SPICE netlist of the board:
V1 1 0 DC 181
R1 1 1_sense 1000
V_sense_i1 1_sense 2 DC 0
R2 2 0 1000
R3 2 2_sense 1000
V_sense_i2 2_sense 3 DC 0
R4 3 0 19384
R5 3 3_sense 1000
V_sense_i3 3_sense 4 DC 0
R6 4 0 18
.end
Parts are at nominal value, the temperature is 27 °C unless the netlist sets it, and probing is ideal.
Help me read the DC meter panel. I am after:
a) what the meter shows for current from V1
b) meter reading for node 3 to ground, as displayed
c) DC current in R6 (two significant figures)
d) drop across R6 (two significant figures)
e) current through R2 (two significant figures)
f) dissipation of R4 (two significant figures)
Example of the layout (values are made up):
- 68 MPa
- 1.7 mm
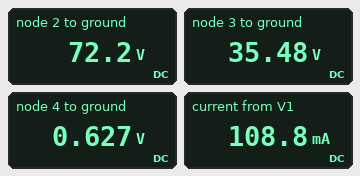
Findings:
- 108.8 mA
- 35.48 V
- 35 mA
- 630 mV
- 72 mA
- 65 mW
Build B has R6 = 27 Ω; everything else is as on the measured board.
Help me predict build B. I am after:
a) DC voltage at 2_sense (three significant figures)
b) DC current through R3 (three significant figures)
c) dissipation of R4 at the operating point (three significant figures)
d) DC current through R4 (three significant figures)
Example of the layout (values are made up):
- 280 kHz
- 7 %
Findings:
- 35.7 V
- 36.6 mA
- 65.6 mW
- 1.84 mA
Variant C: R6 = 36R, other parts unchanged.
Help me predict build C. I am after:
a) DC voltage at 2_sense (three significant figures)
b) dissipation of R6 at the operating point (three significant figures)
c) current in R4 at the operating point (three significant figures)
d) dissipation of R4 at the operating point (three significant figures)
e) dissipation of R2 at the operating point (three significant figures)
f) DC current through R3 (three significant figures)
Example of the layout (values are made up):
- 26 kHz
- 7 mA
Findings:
- 35.8 V
- 43.1 mW
- 1.85 mA
- 66.3 mW
- 5.22 W
- 36.4 mA
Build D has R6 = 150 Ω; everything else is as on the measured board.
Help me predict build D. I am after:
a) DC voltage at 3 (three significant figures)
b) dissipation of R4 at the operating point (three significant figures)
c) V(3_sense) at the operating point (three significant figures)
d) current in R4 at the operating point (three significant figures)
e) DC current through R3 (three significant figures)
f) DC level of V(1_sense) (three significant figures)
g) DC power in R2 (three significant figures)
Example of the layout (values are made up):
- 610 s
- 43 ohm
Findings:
- 38.0 V
- 74.5 mW
- 4.96 V
- 1.96 mA
- 35.0 mA
- 73.0 V
- 5.33 W
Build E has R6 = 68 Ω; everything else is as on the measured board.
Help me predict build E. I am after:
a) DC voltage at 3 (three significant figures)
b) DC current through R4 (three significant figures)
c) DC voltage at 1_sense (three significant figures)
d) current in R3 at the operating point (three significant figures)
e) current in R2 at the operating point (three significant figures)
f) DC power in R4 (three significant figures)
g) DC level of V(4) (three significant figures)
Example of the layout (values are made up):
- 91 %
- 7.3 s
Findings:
- 36.5 V
- 1.88 mA
- 72.5 V
- 36.0 mA
- 72.5 mA
- 68.6 mW
- 2.32 V
